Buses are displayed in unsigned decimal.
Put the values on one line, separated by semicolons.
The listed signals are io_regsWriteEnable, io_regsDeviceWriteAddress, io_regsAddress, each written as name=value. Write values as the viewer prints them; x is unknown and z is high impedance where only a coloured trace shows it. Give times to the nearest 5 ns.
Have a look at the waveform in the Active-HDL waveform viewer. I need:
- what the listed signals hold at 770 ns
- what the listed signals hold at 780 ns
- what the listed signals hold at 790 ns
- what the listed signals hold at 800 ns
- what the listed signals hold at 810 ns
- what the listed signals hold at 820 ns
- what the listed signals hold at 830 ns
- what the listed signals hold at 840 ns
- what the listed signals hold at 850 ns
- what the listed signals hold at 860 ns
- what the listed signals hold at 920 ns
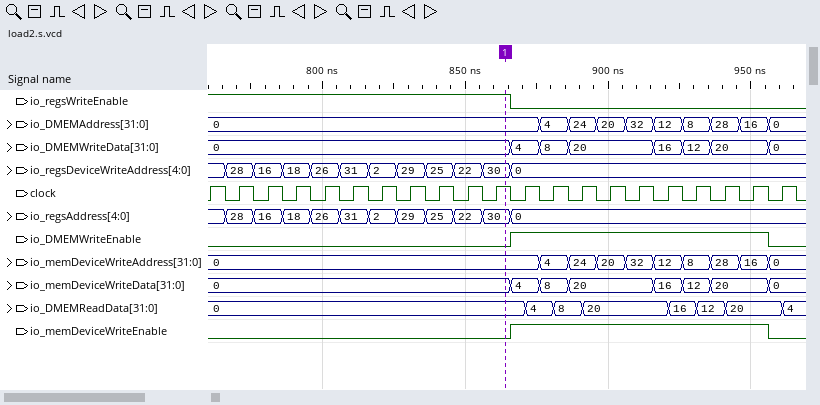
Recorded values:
io_regsWriteEnable=1, io_regsDeviceWriteAddress=28, io_regsAddress=28; io_regsWriteEnable=1, io_regsDeviceWriteAddress=16, io_regsAddress=16; io_regsWriteEnable=1, io_regsDeviceWriteAddress=18, io_regsAddress=18; io_regsWriteEnable=1, io_regsDeviceWriteAddress=26, io_regsAddress=26; io_regsWriteEnable=1, io_regsDeviceWriteAddress=31, io_regsAddress=31; io_regsWriteEnable=1, io_regsDeviceWriteAddress=2, io_regsAddress=2; io_regsWriteEnable=1, io_regsDeviceWriteAddress=29, io_regsAddress=29; io_regsWriteEnable=1, io_regsDeviceWriteAddress=25, io_regsAddress=25; io_regsWriteEnable=1, io_regsDeviceWriteAddress=22, io_regsAddress=22; io_regsWriteEnable=1, io_regsDeviceWriteAddress=30, io_regsAddress=30; io_regsWriteEnable=0, io_regsDeviceWriteAddress=0, io_regsAddress=0
